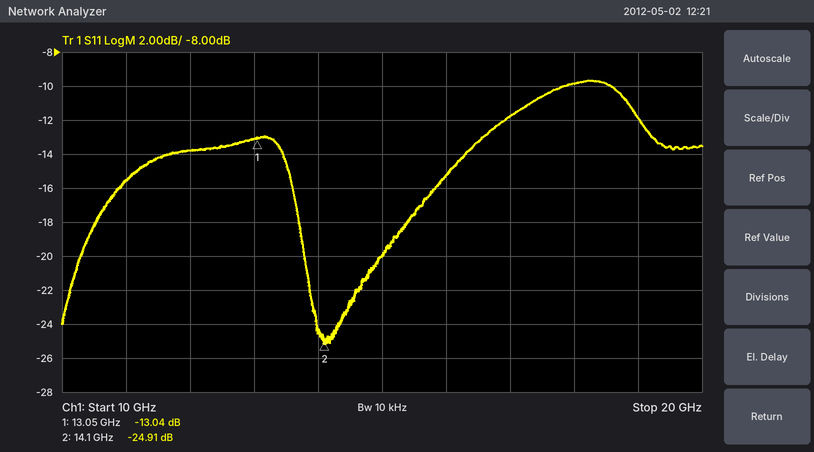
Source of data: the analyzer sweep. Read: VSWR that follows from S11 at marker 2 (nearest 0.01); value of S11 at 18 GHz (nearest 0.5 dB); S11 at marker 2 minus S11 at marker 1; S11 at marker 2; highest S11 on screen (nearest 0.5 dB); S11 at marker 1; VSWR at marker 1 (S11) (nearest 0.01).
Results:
1.12
-10.0 dB
-11.87 dB
-24.91 dB
-9.5 dB
-13.04 dB
1.57
